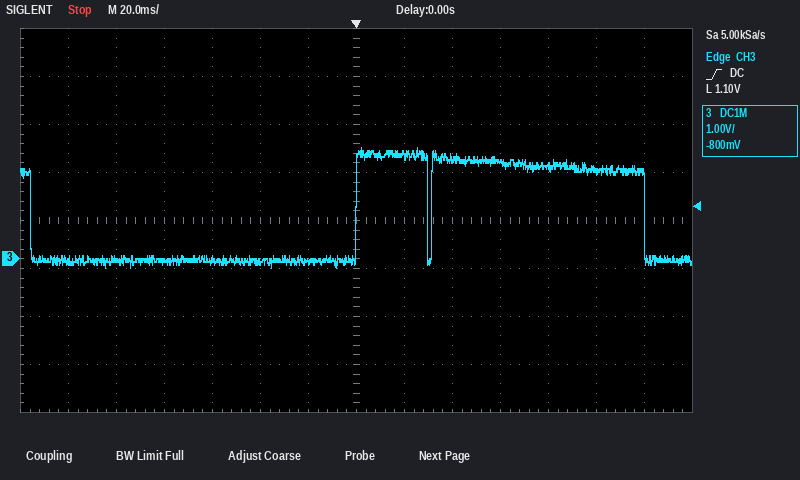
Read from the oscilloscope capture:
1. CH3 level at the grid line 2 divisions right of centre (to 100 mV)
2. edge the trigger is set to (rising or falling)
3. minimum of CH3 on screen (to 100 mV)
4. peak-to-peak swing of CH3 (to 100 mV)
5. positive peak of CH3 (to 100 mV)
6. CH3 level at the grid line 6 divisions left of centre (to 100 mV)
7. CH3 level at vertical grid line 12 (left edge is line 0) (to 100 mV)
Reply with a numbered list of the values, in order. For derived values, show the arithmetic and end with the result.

1. 2.1 V
2. rising
3. -200 mV
4. 2.3 V − (-200 mV) = 2.5 V
5. 2.3 V
6. 0.0 V
7. 1.8 V
